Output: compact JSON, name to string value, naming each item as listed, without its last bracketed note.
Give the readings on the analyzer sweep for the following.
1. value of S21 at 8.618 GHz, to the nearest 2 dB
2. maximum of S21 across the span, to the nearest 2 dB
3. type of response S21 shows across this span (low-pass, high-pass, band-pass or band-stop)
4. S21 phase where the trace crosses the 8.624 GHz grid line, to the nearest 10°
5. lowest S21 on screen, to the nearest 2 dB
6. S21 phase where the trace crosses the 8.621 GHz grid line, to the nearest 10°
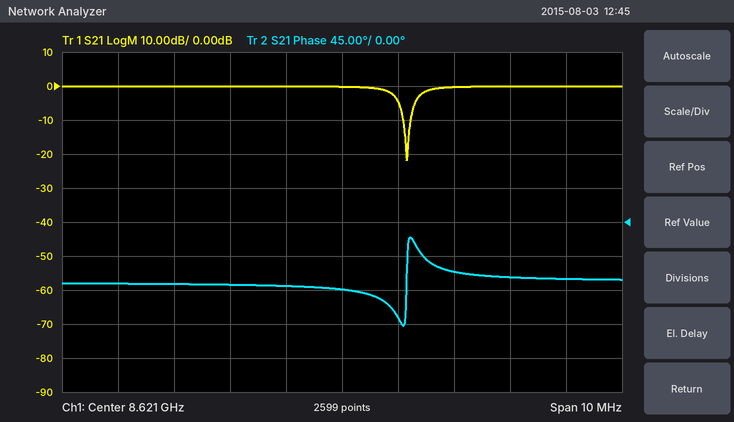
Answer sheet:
{"value of S21 at 8.618 GHz, to the nearest 2 dB": "0 dB", "maximum of S21 across the span, to the nearest 2 dB": "0 dB", "type of response S21 shows across this span": "band-stop", "S21 phase where the trace crosses the 8.624 GHz grid line, to the nearest 10°": "-70°", "lowest S21 on screen, to the nearest 2 dB": "-22 dB", "S21 phase where the trace crosses the 8.621 GHz grid line, to the nearest 10°": "-90°"}
